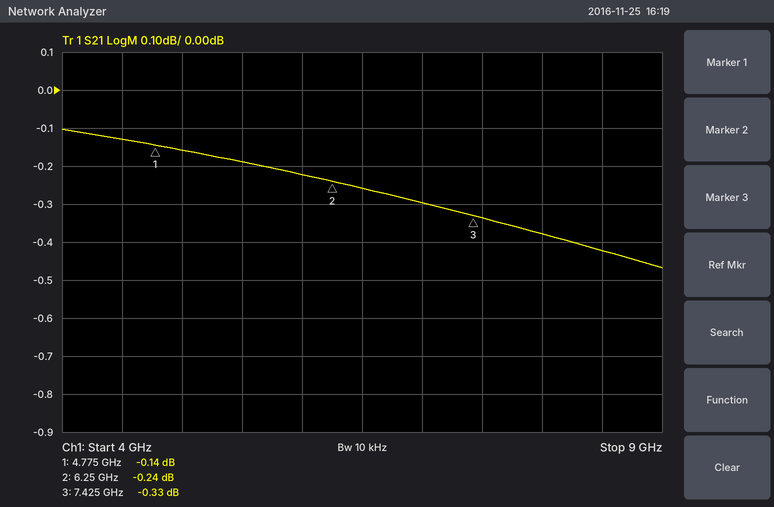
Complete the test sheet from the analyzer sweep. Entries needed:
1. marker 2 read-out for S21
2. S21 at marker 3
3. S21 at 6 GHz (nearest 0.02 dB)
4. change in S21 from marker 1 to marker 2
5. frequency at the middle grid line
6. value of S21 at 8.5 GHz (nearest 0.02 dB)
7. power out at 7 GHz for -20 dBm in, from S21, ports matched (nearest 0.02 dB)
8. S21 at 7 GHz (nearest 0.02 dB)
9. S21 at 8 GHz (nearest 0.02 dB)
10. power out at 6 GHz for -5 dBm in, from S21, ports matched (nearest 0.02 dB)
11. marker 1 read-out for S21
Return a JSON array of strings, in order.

["-0.24 dB", "-0.33 dB", "-0.22 dB", "-0.10 dB", "6.5 GHz", "-0.42 dB", "-20.30 dBm", "-0.30 dB", "-0.38 dB", "-5.22 dBm", "-0.14 dB"]
